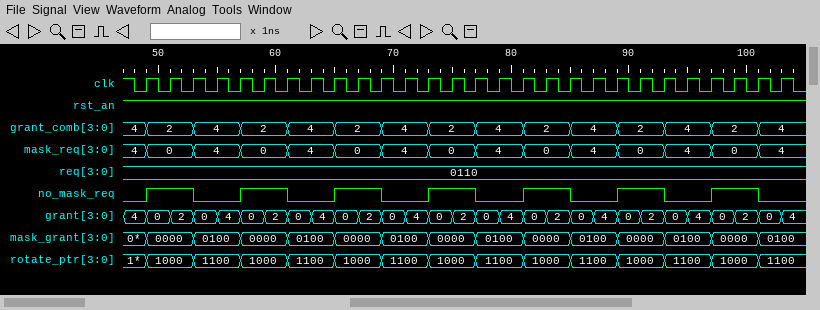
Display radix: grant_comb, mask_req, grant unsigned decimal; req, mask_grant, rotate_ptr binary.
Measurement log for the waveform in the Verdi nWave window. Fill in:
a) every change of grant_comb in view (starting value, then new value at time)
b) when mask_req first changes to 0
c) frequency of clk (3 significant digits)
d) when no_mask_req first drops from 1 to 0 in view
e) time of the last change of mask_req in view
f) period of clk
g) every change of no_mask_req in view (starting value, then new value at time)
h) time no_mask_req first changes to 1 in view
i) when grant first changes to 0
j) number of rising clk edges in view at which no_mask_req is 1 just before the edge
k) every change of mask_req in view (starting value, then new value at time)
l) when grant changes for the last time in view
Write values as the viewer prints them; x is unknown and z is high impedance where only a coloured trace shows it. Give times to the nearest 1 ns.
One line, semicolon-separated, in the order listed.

4, 2 at 49 ns, 4 at 53 ns, 2 at 57 ns, 4 at 61 ns, 2 at 65 ns, 4 at 69 ns, 2 at 73 ns, 4 at 77 ns, 2 at 81 ns, 4 at 85 ns, 2 at 89 ns, 4 at 93 ns, 2 at 97 ns, 4 at 101 ns; 49 ns; 500 MHz; 53 ns; 101 ns; 2 ns; 0, 1 at 49 ns, 0 at 53 ns, 1 at 57 ns, 0 at 61 ns, 1 at 65 ns, 0 at 69 ns, 1 at 73 ns, 0 at 77 ns, 1 at 81 ns, 0 at 85 ns, 1 at 89 ns, 0 at 93 ns, 1 at 97 ns, 0 at 101 ns; 49 ns; 49 ns; 14; 4, 0 at 49 ns, 4 at 53 ns, 0 at 57 ns, 4 at 61 ns, 0 at 65 ns, 4 at 69 ns, 0 at 73 ns, 4 at 77 ns, 0 at 81 ns, 4 at 85 ns, 0 at 89 ns, 4 at 93 ns, 0 at 97 ns, 4 at 101 ns; 103 ns
